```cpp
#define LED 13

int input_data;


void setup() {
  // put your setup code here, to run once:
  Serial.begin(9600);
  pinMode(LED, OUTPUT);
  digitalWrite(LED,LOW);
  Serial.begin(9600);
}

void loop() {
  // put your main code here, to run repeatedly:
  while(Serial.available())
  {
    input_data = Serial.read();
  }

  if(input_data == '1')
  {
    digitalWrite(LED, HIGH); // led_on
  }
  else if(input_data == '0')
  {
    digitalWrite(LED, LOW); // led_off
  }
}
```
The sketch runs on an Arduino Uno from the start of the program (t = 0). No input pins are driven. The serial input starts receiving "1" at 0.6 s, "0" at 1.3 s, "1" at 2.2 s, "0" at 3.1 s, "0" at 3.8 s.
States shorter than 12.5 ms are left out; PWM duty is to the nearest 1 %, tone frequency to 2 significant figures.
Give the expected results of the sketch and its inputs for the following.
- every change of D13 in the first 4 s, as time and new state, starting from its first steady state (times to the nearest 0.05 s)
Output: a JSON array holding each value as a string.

["0 s low; 0.6 s high; 1.3 s low; 2.2 s high; 3.1 s low"]
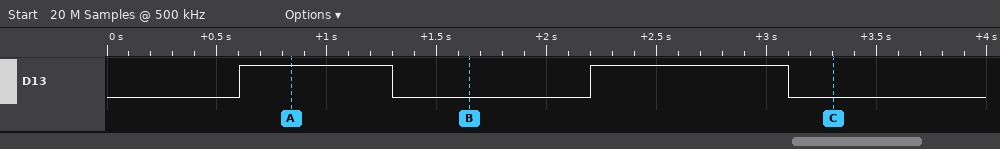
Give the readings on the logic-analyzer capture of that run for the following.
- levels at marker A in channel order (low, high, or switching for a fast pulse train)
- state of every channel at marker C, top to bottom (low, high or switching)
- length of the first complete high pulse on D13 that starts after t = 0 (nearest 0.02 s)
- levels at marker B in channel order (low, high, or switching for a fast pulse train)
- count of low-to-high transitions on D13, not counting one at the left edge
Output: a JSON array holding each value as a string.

["D13 high", "D13 low", "0.70 s", "D13 low", "2"]
